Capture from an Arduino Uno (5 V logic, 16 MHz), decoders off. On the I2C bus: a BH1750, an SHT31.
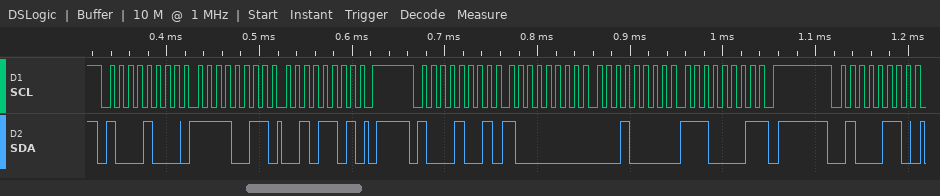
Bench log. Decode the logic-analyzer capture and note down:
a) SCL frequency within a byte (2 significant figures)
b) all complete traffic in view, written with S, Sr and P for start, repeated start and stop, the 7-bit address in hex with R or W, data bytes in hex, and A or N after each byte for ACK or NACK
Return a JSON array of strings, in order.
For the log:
["100 kHz", "S 44W A F3 A 2D A P S 44R A 80 A 10 A E1 N P S 23W A"]
